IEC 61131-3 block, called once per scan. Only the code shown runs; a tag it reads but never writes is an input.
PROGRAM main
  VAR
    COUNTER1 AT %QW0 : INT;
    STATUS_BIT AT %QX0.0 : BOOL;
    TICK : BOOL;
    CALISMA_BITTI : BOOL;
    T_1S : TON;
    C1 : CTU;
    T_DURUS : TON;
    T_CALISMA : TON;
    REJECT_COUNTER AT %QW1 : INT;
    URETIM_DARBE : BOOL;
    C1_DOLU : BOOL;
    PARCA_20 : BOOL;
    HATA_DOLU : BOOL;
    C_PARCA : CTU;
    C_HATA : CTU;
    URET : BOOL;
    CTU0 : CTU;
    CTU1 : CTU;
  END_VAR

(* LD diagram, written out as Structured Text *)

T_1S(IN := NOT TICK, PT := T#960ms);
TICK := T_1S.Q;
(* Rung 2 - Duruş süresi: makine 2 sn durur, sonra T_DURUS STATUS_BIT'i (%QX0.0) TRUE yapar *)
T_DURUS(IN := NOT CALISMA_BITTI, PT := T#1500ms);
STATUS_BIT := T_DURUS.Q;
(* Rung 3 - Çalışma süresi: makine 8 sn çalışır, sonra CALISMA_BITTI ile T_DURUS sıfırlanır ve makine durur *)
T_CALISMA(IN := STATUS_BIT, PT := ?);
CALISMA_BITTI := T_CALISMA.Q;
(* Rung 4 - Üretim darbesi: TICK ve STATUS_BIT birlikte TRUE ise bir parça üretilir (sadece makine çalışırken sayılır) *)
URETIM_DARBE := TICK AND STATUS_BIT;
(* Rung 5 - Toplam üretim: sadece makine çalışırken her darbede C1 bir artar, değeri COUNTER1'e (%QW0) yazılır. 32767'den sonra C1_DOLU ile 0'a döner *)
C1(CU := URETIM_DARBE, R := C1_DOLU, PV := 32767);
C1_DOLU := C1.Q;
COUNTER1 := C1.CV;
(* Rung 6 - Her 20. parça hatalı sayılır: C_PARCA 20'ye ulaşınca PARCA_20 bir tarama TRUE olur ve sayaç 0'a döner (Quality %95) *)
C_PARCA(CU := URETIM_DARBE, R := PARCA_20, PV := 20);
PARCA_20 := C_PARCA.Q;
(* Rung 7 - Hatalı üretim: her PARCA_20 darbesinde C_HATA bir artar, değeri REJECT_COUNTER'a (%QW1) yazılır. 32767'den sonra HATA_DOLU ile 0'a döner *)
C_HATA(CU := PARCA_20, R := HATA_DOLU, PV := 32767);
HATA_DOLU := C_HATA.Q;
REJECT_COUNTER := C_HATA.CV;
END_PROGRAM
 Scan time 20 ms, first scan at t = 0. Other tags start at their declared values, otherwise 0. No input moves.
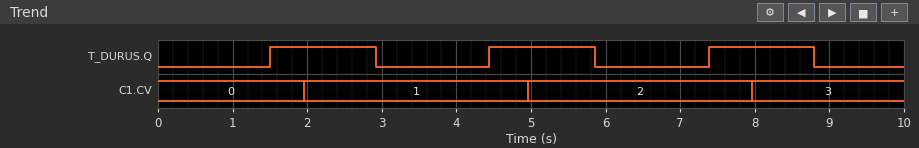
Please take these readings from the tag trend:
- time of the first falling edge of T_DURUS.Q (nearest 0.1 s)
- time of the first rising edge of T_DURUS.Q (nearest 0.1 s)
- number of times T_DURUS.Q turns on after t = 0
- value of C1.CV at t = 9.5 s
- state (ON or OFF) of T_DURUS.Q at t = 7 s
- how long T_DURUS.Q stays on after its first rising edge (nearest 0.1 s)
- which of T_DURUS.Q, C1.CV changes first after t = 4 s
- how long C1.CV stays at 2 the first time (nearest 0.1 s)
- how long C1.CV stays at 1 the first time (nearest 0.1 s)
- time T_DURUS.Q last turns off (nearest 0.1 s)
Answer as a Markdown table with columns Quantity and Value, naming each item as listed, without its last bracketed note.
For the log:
| Quantity | Value |
|---|---|
| time of the first falling edge of T_DURUS.Q | 2.9 s |
| time of the first rising edge of T_DURUS.Q | 1.5 s |
| number of times T_DURUS.Q turns on after t = 0 | 3 |
| value of C1.CV at t = 9.5 s | 3 |
| state (ON or OFF) of T_DURUS.Q at t = 7 s | OFF |
| how long T_DURUS.Q stays on after its first rising edge | 1.4 s |
| which of T_DURUS.Q, C1.CV changes first after t = 4 s | T_DURUS.Q |
| how long C1.CV stays at 2 the first time | 3.0 s |
| how long C1.CV stays at 1 the first time | 3.0 s |
| time T_DURUS.Q last turns off | 8.8 s |
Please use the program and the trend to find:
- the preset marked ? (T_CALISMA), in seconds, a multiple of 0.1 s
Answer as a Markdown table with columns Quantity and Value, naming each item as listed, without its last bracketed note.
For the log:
| Quantity | Value |
|---|---|
| the preset marked ? (T_CALISMA), in seconds, a multiple of 0.1 s | 1.4 s |
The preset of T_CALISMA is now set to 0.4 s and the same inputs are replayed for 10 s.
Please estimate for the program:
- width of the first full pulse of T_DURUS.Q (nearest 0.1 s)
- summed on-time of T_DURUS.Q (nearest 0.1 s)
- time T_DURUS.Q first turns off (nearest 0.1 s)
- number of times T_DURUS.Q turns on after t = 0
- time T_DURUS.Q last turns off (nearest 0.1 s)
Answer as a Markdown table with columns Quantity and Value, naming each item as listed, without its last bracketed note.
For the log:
| Quantity | Value |
|---|---|
| width of the first full pulse of T_DURUS.Q | 0.4 s |
| summed on-time of T_DURUS.Q | 2.1 s |
| time T_DURUS.Q first turns off | 1.9 s |
| number of times T_DURUS.Q turns on after t = 0 | 5 |
| time T_DURUS.Q last turns off | 9.7 s |
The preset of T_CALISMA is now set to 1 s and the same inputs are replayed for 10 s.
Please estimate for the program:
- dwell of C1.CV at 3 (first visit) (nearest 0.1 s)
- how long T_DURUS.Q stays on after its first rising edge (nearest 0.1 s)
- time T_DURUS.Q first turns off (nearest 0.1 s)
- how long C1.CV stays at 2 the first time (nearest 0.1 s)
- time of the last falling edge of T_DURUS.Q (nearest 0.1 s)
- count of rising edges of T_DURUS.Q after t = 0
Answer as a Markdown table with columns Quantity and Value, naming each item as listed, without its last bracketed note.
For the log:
| Quantity | Value |
|---|---|
| dwell of C1.CV at 3 (first visit) | 3.0 s |
| how long T_DURUS.Q stays on after its first rising edge | 1.0 s |
| time T_DURUS.Q first turns off | 2.5 s |
| how long C1.CV stays at 2 the first time | 2.0 s |
| time of the last falling edge of T_DURUS.Q | 7.6 s |
| count of rising edges of T_DURUS.Q after t = 0 | 4 |
